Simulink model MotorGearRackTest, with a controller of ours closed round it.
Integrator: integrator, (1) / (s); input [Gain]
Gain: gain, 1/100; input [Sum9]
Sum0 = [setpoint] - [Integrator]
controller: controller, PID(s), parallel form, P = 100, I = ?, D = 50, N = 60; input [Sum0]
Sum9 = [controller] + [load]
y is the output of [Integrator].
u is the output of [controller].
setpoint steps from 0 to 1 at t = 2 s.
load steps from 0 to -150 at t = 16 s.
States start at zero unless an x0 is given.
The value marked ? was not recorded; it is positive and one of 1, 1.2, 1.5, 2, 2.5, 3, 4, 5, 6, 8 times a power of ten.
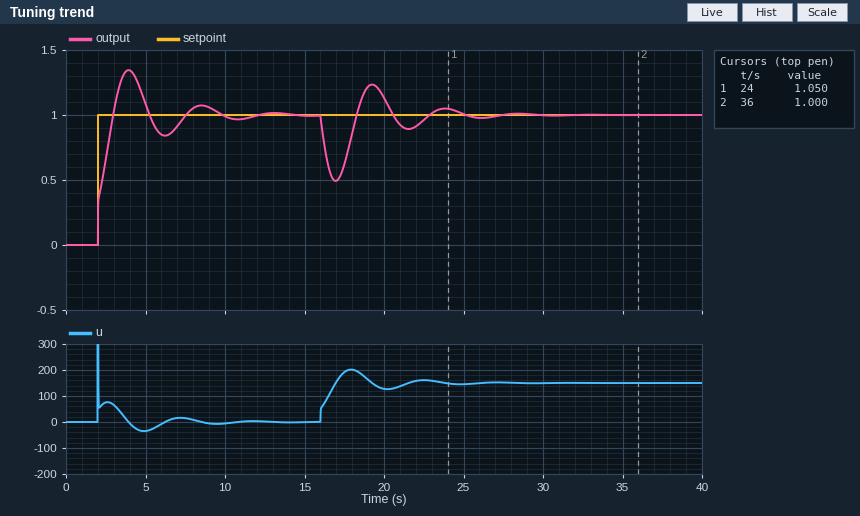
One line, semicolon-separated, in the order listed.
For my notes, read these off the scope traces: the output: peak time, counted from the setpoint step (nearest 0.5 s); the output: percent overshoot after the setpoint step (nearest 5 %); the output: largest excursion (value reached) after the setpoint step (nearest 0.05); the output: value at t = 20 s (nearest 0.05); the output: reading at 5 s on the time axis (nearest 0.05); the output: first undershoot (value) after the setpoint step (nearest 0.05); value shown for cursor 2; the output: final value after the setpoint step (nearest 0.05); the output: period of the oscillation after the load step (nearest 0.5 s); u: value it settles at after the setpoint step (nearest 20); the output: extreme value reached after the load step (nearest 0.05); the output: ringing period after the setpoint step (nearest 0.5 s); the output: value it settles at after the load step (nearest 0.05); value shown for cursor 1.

2.0 s; 35 %; 1.35; 1.15; 1.10; 0.85; 1.000; 1.00; 4.5 s; 0; 0.50; 4.5 s; 1.00; 1.050
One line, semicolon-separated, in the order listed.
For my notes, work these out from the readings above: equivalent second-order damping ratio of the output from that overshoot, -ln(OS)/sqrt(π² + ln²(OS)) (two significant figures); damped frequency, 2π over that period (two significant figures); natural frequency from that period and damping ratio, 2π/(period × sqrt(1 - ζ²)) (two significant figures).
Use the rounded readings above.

0.32; 1.4 rad/s; 1.5 rad/s
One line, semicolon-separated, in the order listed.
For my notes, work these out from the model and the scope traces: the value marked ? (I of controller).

300
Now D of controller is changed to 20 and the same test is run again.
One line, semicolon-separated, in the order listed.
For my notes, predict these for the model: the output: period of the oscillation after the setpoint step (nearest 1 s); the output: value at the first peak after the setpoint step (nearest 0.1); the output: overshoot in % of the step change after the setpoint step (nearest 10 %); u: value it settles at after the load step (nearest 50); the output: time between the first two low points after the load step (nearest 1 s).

4 s; 1.4; 40 %; 150; 4 s
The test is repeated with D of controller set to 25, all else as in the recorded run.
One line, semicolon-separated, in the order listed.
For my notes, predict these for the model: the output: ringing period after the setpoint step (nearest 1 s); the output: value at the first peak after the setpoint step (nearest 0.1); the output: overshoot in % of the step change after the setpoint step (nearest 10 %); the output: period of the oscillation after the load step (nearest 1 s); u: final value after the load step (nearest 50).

4 s; 1.4; 40 %; 4 s; 150
